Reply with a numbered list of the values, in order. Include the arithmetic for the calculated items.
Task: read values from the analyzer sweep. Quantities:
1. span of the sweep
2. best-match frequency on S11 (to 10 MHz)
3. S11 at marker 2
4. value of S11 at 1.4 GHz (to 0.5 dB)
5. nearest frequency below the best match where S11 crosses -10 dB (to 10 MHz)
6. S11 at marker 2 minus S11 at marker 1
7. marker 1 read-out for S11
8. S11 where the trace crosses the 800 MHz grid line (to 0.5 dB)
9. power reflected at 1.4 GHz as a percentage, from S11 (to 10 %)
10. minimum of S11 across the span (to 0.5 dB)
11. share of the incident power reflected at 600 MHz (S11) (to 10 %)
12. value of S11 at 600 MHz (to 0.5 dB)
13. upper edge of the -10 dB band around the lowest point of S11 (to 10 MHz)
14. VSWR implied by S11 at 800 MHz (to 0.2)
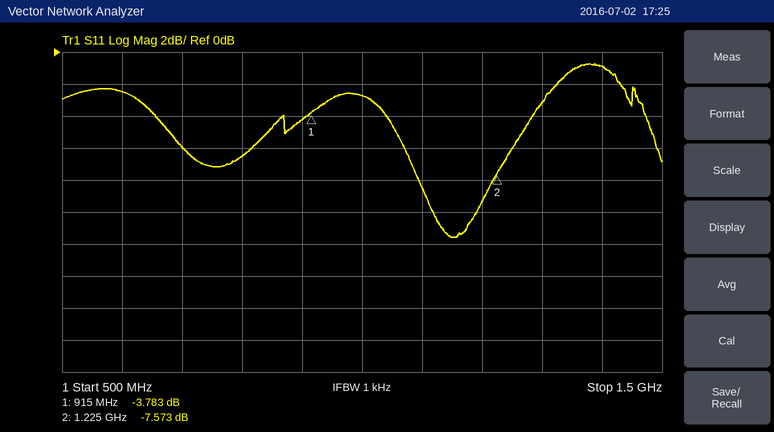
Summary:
1. 1 GHz
2. 1.15 GHz
3. -7.573 dB
4. -1.0 dB
5. 1.12 GHz
6. -7.573 − (-3.783) = -3.790 dB
7. -3.783 dB
8. -6.5 dB
9. 10^(-1/10) ≈ 79.4 %, so 80 % to the nearest 10 %
10. -11.5 dB
11. 10^(-2.5/10) ≈ 56.2 %, so 60 % to the nearest 10 %
12. -2.5 dB
13. 1.19 GHz
14. |Γ| = 10^(-6.5/20) = 0.4732; VSWR = (1 + 0.4732)/(1 − 0.4732) ≈ 2.8
